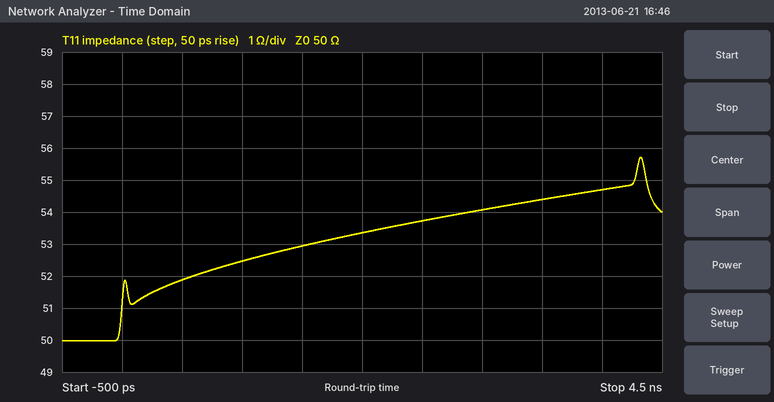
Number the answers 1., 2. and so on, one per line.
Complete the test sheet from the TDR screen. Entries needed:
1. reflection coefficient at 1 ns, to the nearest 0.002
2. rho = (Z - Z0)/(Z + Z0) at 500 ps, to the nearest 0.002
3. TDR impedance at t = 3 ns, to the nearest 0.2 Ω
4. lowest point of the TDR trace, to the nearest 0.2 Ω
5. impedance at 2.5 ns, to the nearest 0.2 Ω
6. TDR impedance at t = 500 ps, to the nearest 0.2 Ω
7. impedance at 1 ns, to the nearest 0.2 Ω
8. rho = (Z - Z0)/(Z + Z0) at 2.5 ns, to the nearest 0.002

1. +0.024
2. +0.018
3. 54.0 Ω
4. 50.0 Ω
5. 53.8 Ω
6. 51.8 Ω
7. 52.4 Ω
8. +0.036
